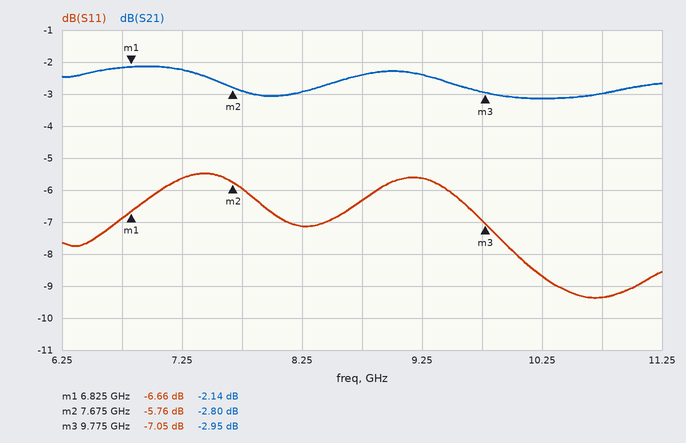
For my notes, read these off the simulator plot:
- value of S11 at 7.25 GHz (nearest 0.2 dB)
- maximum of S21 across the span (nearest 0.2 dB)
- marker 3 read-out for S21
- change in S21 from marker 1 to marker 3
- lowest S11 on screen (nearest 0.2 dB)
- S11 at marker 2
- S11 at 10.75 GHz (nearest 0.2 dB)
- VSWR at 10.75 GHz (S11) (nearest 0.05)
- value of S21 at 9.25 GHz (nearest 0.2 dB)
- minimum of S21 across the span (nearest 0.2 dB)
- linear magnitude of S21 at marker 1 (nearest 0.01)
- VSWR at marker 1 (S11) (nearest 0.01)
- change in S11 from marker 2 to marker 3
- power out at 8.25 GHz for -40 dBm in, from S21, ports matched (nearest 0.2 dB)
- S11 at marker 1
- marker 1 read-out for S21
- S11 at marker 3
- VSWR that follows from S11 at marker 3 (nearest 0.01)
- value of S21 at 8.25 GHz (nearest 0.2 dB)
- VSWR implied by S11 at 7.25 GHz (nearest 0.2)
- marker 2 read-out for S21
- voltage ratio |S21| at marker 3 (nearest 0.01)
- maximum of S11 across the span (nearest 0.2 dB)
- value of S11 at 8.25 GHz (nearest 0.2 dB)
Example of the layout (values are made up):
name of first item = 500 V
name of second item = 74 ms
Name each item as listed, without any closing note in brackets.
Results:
value of S11 at 7.25 GHz = -5.6 dB
maximum of S21 across the span = -2.2 dB
marker 3 read-out for S21 = -2.95 dB
change in S21 from marker 1 to marker 3 = -0.81 dB
lowest S11 on screen = -9.4 dB
S11 at marker 2 = -5.76 dB
S11 at 10.75 GHz = -9.4 dB
VSWR at 10.75 GHz (S11) = 2.05
value of S21 at 9.25 GHz = -2.4 dB
minimum of S21 across the span = -3.2 dB
linear magnitude of S21 at marker 1 = 0.78
VSWR at marker 1 (S11) = 2.73
change in S11 from marker 2 to marker 3 = -1.29 dB
power out at 8.25 GHz for -40 dBm in, from S21, ports matched = -43.0 dBm
S11 at marker 1 = -6.66 dB
marker 1 read-out for S21 = -2.14 dB
S11 at marker 3 = -7.05 dB
VSWR that follows from S11 at marker 3 = 2.60
value of S21 at 8.25 GHz = -3.0 dB
VSWR implied by S11 at 7.25 GHz = 3.2
marker 2 read-out for S21 = -2.80 dB
voltage ratio |S21| at marker 3 = 0.71
maximum of S11 across the span = -5.4 dB
value of S11 at 8.25 GHz = -7.2 dB
